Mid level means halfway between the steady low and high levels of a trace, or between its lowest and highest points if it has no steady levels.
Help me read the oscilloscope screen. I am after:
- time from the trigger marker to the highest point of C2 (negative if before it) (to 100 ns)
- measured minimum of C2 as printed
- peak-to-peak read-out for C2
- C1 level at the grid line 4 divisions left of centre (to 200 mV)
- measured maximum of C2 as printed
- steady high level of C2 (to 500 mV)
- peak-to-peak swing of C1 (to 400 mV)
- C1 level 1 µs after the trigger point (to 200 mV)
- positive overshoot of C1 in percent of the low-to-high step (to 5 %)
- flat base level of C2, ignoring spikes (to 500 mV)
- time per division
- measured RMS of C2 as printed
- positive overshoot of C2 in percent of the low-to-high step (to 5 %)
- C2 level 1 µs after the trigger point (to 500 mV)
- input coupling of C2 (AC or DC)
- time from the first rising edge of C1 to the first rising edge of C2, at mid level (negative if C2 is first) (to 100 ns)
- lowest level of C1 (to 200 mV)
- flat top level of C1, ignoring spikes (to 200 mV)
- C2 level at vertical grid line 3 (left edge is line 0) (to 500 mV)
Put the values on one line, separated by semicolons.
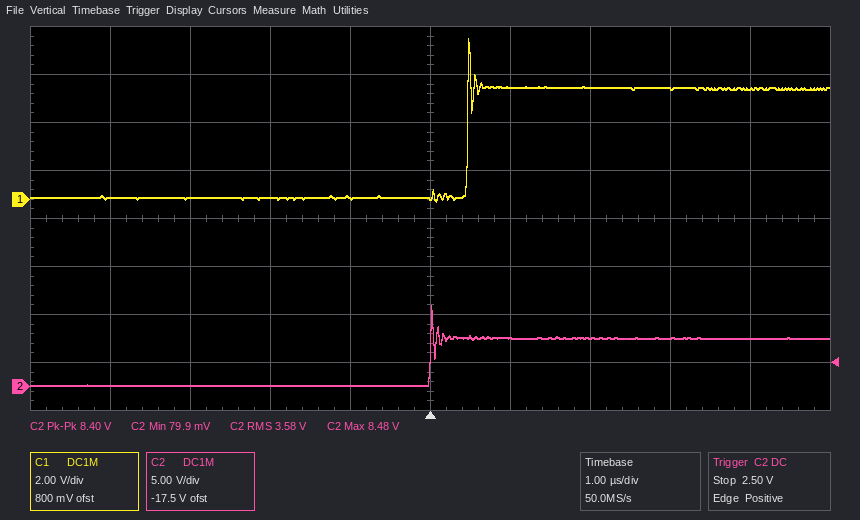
0.0 µs; 79.9 mV; 8.40 V; 0.0 V; 8.48 V; 5.0 V; 6.8 V; 4.6 V; 45 %; 0.0 V; 1 µs; 3.58 V; 70 %; 5.0 V; DC; -500 ns; 0.0 V; 4.6 V; 0.0 V
